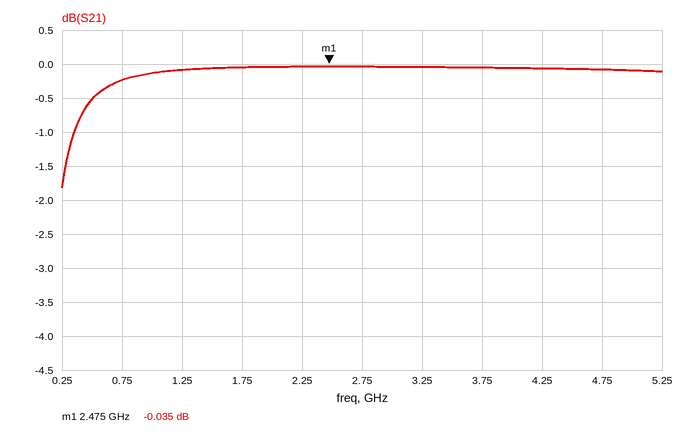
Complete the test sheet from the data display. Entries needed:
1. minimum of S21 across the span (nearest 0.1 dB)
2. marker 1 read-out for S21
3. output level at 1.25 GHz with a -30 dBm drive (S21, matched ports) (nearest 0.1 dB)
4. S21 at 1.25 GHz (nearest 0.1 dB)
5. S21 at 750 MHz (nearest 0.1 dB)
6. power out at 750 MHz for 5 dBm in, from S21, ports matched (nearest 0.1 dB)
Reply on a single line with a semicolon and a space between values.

-1.8 dB; -0.035 dB; -30.1 dBm; -0.1 dB; -0.2 dB; 4.8 dBm
